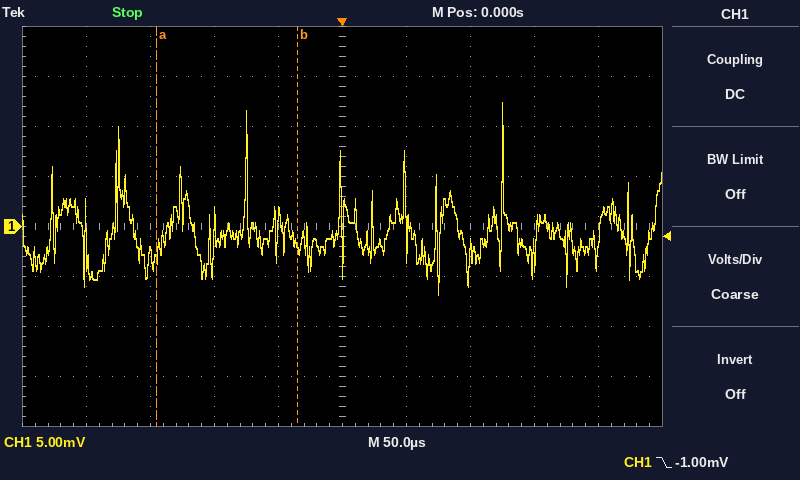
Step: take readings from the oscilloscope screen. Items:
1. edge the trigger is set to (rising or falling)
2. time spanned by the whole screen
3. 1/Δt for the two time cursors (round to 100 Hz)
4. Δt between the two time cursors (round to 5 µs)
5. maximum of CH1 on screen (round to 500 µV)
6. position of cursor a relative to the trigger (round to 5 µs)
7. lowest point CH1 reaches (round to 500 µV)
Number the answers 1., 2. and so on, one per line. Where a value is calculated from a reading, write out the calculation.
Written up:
1. falling
2. 500 µs
3. 1 / 110 µs ≈ 9.1 kHz
4. 110 µs
5. 12.5 mV
6. -145 µs
7. -7.0 mV
